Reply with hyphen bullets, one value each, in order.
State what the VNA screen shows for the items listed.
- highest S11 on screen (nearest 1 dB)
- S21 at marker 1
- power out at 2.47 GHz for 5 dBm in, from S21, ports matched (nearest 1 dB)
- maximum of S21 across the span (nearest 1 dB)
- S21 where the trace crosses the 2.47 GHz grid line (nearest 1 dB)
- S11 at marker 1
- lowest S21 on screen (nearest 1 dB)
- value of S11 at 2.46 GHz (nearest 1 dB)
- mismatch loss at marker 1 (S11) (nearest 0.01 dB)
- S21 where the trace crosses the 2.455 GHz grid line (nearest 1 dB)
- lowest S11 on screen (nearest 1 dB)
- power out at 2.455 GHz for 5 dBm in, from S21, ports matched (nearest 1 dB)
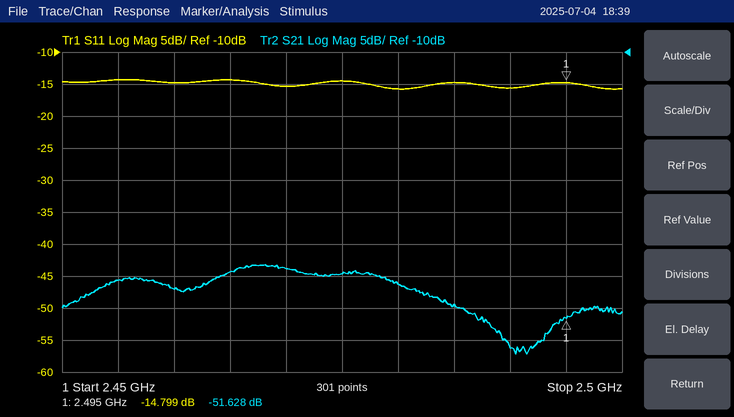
- -14 dB
- -51.628 dB
- -39 dBm
- -43 dB
- -44 dB
- -14.799 dB
- -57 dB
- -15 dB
- 0.15 dB
- -46 dB
- -16 dB
- -41 dBm
